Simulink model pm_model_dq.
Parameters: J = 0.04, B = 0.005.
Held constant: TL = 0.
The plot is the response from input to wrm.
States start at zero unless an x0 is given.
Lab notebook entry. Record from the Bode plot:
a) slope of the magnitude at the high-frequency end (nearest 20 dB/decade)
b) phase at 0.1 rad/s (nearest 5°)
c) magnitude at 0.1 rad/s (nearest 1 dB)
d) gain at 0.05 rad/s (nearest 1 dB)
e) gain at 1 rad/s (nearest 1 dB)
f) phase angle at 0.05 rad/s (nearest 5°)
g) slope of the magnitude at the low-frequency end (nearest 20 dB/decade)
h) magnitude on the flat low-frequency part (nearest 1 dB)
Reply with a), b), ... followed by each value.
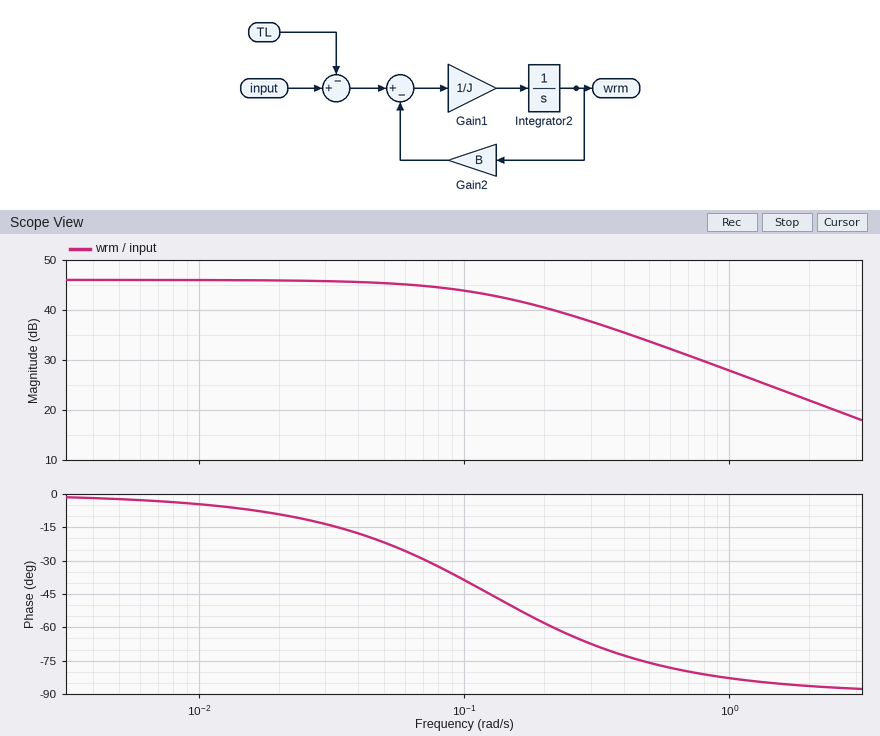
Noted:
a) -20 dB/decade
b) -40°
c) 44 dB
d) 45 dB
e) 28 dB
f) -20°
g) 0 dB/decade
h) 46 dB
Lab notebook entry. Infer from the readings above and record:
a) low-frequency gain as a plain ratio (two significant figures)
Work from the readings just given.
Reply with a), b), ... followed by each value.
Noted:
a) 200
